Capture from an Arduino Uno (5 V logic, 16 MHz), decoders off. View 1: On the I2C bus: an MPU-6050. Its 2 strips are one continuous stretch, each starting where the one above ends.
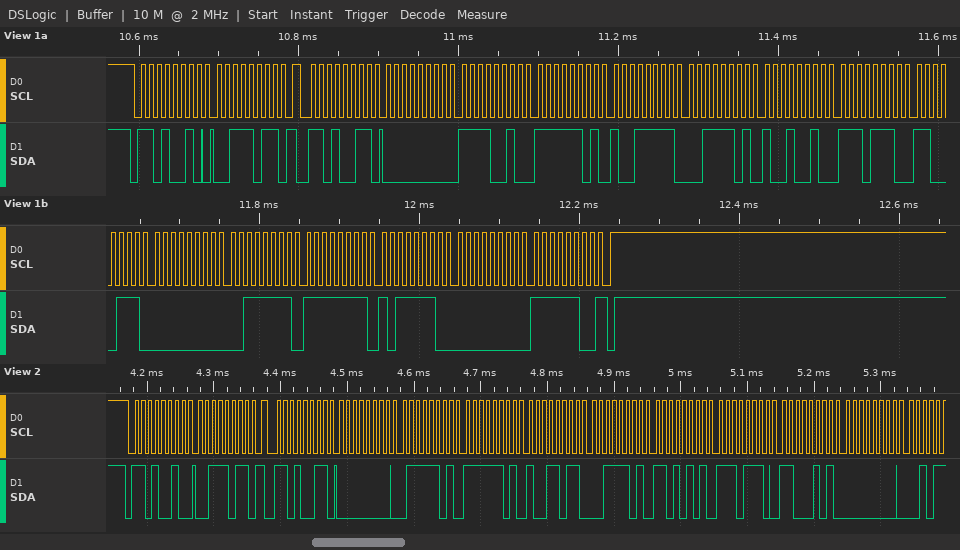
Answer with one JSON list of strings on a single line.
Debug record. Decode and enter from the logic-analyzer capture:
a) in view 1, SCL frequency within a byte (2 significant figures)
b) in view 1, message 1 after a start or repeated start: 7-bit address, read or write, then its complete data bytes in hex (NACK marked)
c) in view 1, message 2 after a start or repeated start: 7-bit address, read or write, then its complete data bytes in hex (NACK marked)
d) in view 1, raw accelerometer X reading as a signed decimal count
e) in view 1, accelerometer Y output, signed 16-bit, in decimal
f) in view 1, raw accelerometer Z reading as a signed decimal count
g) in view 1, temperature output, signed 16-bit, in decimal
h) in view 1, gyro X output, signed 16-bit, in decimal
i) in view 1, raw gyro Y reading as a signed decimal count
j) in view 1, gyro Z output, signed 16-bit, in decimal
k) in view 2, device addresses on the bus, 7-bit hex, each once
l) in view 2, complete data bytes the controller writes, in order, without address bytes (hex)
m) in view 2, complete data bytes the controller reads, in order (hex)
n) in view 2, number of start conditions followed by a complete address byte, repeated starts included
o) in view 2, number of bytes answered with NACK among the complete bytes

["100 kHz", "0x69 write: 3B", "0x69 read: 00 F2 FD 9F 3D 92 EE C7 00 3F FF BE 00 FC NACK", "242", "-609", "15762", "-4409", "63", "-66", "252", "0x69", "3B", "00 7D FD 9B 3D D5 EE C5 00", "2", "0"]
